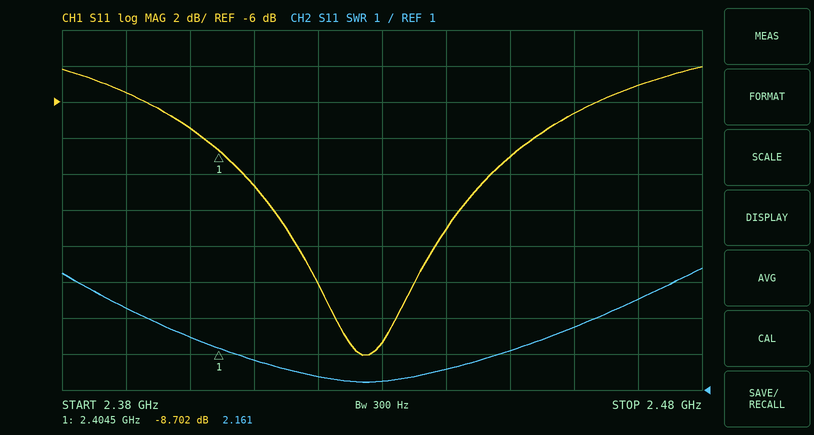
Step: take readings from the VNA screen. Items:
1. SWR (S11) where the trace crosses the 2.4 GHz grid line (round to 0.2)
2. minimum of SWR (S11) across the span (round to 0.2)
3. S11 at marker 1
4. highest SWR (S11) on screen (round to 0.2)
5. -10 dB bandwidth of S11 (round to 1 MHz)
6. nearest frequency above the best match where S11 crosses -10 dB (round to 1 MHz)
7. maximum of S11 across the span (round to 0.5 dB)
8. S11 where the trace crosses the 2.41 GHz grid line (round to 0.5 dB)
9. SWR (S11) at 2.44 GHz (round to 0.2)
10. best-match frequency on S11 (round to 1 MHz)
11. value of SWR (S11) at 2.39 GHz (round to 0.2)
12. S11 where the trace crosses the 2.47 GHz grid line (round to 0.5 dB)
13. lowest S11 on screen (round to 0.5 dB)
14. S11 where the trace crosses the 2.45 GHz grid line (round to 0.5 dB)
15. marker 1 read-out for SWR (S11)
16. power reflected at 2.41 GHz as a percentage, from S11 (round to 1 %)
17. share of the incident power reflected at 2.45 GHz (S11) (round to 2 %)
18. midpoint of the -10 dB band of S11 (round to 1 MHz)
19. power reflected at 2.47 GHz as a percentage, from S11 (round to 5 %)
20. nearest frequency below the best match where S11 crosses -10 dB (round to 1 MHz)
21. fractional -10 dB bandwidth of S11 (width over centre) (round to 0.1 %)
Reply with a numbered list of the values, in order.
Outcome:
1. 2.4
2. 1.2
3. -8.702 dB
4. 4.4
5. 39 MHz
6. 2.447 GHz
7. -4.0 dB
8. -10.5 dB
9. 1.6
10. 2.427 GHz
11. 3.2
12. -5.0 dB
13. -20.0 dB
14. -9.0 dB
15. 2.161
16. 9 %
17. 12 %
18. 2.428 GHz
19. 30 %
20. 2.408 GHz
21. 1.6 %
